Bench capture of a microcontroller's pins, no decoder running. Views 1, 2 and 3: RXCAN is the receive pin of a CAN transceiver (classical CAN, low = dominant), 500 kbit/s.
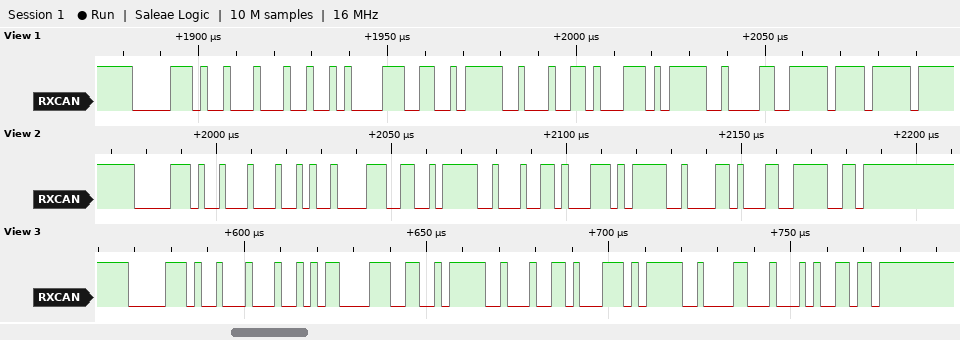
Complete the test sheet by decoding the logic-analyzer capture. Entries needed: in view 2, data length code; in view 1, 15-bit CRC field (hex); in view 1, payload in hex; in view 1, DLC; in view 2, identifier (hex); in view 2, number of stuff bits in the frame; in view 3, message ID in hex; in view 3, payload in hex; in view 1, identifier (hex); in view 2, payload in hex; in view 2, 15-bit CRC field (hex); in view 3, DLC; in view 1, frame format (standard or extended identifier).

8
0x3FEF
92 87 32 FA 26 8E BE 86
8
0x069
4
0x069
95 87 32 FA 26 8E BE 86
0x069
94 87 32 FA 26 8E BE 86
0x467D
8
standard
